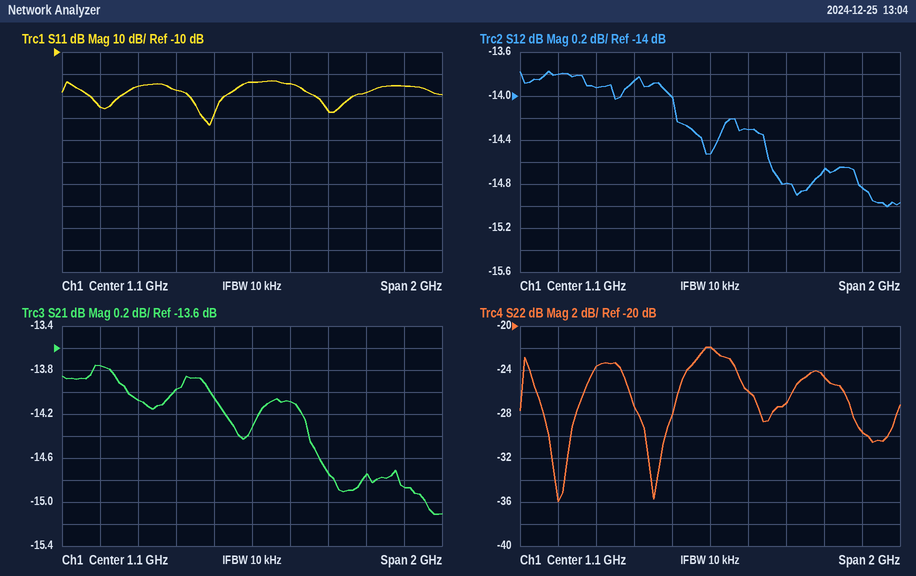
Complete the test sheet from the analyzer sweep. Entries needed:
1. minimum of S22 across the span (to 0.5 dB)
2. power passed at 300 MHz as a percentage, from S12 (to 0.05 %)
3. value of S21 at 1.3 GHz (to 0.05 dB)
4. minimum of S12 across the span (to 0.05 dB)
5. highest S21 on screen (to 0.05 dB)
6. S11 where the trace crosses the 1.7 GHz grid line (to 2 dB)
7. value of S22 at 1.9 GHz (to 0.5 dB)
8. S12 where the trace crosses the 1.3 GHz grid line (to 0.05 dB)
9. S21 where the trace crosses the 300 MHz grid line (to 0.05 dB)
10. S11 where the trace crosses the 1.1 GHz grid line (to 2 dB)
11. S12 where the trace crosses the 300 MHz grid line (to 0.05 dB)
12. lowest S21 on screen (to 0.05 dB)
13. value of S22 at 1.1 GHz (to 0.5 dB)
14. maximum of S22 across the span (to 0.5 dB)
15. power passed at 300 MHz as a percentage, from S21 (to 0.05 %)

-36.0 dB
4.15 %
-14.10 dB
-15.00 dB
-13.75 dB
-28 dB
-29.5 dB
-14.30 dB
-13.75 dB
-24 dB
-13.80 dB
-15.10 dB
-22.0 dB
-22.0 dB
4.20 %
